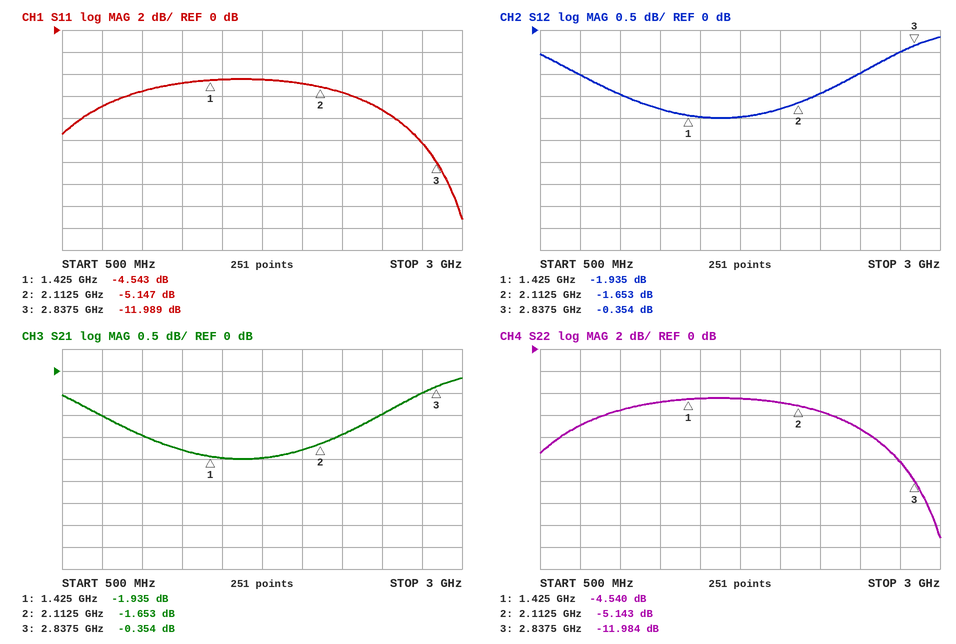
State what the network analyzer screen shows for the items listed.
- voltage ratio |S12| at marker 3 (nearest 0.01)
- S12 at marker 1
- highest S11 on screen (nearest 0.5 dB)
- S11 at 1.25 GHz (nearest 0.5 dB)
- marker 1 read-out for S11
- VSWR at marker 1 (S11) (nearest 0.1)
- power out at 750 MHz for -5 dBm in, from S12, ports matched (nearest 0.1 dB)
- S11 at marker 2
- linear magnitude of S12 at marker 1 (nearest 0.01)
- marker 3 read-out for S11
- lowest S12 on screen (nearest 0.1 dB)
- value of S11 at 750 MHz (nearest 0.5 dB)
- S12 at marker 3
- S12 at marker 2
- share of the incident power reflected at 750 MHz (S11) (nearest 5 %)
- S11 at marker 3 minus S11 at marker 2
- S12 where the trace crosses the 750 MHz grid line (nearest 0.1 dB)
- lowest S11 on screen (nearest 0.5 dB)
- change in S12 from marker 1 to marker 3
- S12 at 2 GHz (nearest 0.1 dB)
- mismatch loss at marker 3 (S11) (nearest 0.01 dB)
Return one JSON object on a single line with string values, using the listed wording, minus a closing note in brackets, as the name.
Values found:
{"voltage ratio |S12| at marker 3": "0.96", "S12 at marker 1": "-1.935 dB", "highest S11 on screen": "-4.5 dB", "S11 at 1.25 GHz": "-5.0 dB", "marker 1 read-out for S11": "-4.543 dB", "VSWR at marker 1 (S11)": "3.9", "power out at 750 MHz for -5 dBm in, from S12, ports matched": "-6.0 dBm", "S11 at marker 2": "-5.147 dB", "linear magnitude of S12 at marker 1": "0.80", "marker 3 read-out for S11": "-11.989 dB", "lowest S12 on screen": "-2.0 dB", "value of S11 at 750 MHz": "-7.0 dB", "S12 at marker 3": "-0.354 dB", "S12 at marker 2": "-1.653 dB", "share of the incident power reflected at 750 MHz (S11)": "20 %", "S11 at marker 3 minus S11 at marker 2": "-6.842 dB", "S12 where the trace crosses the 750 MHz grid line": "-1.0 dB", "lowest S11 on screen": "-17.0 dB", "change in S12 from marker 1 to marker 3": "1.581 dB", "S12 at 2 GHz": "-1.8 dB", "mismatch loss at marker 3 (S11)": "0.28 dB"}
